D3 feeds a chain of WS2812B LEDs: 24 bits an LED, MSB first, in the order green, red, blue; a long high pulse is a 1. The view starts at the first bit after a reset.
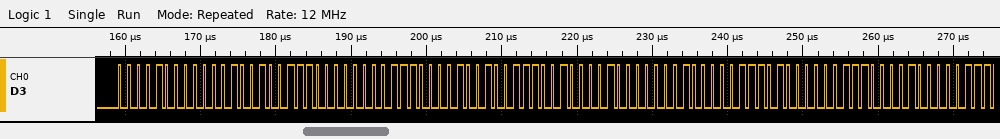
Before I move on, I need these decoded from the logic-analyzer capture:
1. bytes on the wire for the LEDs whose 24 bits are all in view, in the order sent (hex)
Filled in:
08 09 38 07 09 39 08 08 3A
